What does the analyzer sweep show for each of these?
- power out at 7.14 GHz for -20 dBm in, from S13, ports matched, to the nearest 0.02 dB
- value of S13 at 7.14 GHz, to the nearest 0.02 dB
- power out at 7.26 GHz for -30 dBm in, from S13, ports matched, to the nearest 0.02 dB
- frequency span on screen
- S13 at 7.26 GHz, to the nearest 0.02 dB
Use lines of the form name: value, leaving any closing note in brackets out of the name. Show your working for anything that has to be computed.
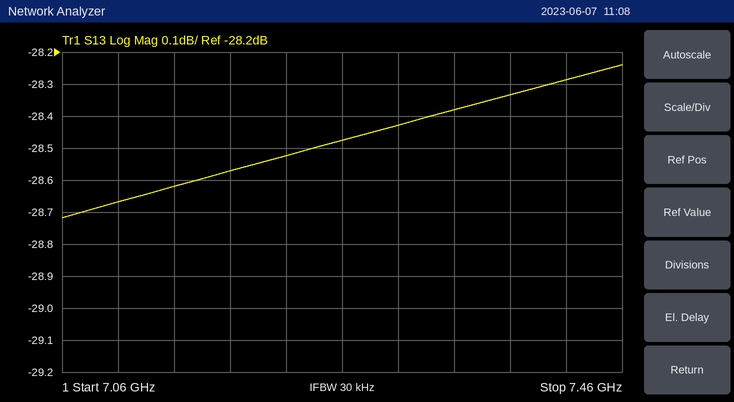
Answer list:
power out at 7.14 GHz for -20 dBm in, from S13, ports matched, to the nearest 0.02 dB: -20 dBm + (-28.62 dB) = -48.62 dBm
value of S13 at 7.14 GHz, to the nearest 0.02 dB: -28.62 dB
power out at 7.26 GHz for -30 dBm in, from S13, ports matched, to the nearest 0.02 dB: -30 dBm + (-28.48 dB) = -58.48 dBm
frequency span on screen: 400 MHz
S13 at 7.26 GHz, to the nearest 0.02 dB: -28.48 dB
